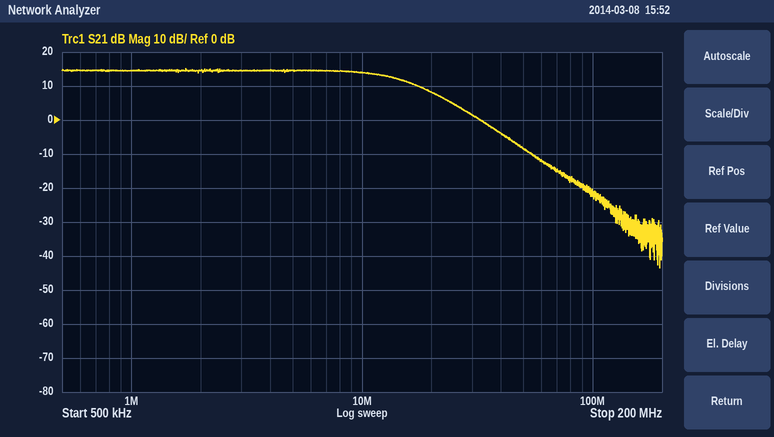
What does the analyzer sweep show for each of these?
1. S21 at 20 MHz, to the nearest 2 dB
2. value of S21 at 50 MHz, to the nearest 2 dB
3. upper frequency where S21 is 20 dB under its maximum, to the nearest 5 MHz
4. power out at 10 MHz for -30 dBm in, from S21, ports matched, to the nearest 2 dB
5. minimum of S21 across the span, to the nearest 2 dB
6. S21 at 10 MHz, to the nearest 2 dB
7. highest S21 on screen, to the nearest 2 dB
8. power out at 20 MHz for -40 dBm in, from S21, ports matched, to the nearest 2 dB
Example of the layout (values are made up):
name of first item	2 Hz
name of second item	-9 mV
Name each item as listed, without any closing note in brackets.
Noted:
S21 at 20 MHz, to the nearest 2 dB	8 dB
value of S21 at 50 MHz, to the nearest 2 dB	-8 dB
upper frequency where S21 is 20 dB under its maximum, to the nearest 5 MHz	40 MHz
power out at 10 MHz for -30 dBm in, from S21, ports matched, to the nearest 2 dB	-16 dBm
minimum of S21 across the span, to the nearest 2 dB	-44 dB
S21 at 10 MHz, to the nearest 2 dB	14 dB
highest S21 on screen, to the nearest 2 dB	16 dB
power out at 20 MHz for -40 dBm in, from S21, ports matched, to the nearest 2 dB	-32 dBm
